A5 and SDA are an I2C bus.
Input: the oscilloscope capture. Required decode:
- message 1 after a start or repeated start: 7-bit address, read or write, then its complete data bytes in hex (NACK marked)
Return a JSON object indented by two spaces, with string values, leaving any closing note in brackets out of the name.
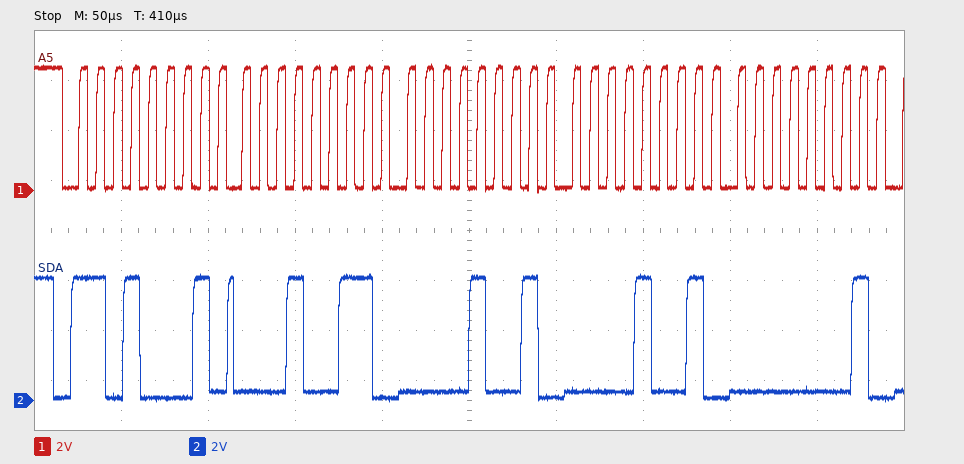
{
  "message 1 after a start or repeated start: 7-bit address, read or write, then its complete data bytes in hex": "0x68 read: 13 09 09 01"
}
